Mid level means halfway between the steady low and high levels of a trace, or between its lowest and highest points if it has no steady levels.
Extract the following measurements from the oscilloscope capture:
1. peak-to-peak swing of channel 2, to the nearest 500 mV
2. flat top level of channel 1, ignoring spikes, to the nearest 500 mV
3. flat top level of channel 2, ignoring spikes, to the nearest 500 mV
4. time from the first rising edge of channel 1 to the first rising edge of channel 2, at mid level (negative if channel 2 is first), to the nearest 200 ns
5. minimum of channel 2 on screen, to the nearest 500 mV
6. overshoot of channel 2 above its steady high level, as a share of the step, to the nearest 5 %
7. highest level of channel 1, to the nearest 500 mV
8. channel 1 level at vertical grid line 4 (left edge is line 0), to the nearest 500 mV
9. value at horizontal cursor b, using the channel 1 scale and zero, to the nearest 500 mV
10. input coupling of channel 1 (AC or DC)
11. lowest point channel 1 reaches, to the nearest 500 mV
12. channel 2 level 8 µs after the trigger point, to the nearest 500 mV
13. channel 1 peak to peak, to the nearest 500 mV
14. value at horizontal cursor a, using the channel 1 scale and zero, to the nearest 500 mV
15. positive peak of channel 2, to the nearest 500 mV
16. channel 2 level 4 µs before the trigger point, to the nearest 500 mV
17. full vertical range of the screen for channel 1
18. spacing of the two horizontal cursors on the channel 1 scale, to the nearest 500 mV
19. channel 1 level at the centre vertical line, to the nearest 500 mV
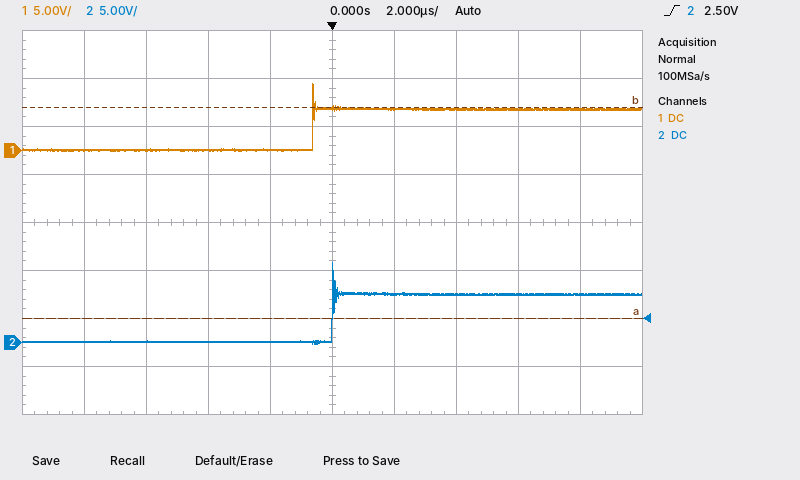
8.5 V
4.5 V
5.0 V
+600 ns
0.0 V
65 %
7.0 V
0.0 V
4.5 V
DC
0.0 V
5.0 V
7.0 V
-17.5 V
8.5 V
0.0 V
40 V
22.0 V
4.5 V
